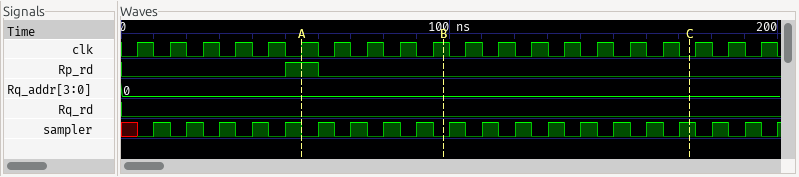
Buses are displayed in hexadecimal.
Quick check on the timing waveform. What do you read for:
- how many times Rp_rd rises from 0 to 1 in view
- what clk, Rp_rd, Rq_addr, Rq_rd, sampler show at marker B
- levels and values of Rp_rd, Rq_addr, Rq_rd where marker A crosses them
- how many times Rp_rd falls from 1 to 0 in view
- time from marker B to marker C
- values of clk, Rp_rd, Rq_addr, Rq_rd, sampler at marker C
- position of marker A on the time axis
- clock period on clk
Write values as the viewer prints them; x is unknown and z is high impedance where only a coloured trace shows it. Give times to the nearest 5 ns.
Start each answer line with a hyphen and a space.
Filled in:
- 1
- clk=1, Rp_rd=0, Rq_addr=0, Rq_rd=0, sampler=0
- Rp_rd=1, Rq_addr=0, Rq_rd=0
- 1
- 75 ns
- clk=0, Rp_rd=0, Rq_addr=0, Rq_rd=0, sampler=1
- 55 ns
- 10 ns
